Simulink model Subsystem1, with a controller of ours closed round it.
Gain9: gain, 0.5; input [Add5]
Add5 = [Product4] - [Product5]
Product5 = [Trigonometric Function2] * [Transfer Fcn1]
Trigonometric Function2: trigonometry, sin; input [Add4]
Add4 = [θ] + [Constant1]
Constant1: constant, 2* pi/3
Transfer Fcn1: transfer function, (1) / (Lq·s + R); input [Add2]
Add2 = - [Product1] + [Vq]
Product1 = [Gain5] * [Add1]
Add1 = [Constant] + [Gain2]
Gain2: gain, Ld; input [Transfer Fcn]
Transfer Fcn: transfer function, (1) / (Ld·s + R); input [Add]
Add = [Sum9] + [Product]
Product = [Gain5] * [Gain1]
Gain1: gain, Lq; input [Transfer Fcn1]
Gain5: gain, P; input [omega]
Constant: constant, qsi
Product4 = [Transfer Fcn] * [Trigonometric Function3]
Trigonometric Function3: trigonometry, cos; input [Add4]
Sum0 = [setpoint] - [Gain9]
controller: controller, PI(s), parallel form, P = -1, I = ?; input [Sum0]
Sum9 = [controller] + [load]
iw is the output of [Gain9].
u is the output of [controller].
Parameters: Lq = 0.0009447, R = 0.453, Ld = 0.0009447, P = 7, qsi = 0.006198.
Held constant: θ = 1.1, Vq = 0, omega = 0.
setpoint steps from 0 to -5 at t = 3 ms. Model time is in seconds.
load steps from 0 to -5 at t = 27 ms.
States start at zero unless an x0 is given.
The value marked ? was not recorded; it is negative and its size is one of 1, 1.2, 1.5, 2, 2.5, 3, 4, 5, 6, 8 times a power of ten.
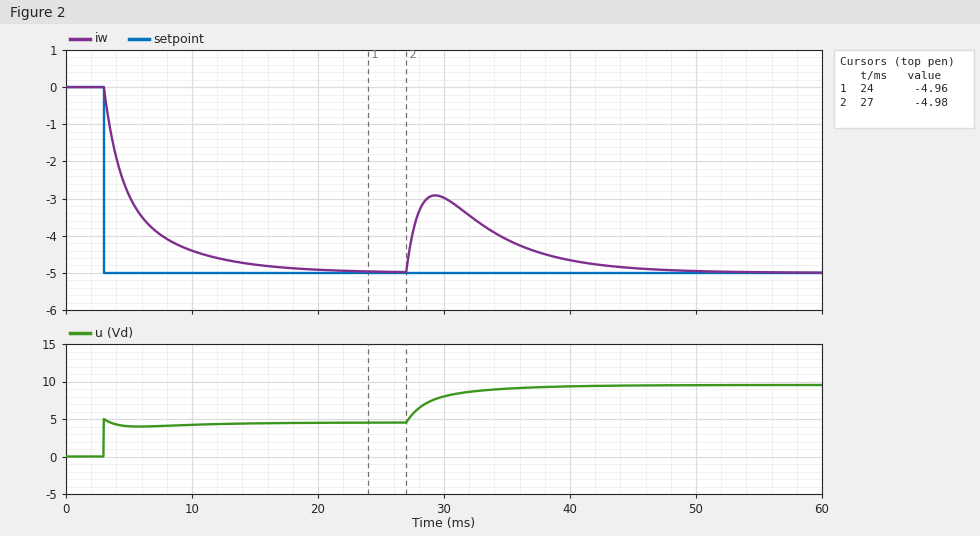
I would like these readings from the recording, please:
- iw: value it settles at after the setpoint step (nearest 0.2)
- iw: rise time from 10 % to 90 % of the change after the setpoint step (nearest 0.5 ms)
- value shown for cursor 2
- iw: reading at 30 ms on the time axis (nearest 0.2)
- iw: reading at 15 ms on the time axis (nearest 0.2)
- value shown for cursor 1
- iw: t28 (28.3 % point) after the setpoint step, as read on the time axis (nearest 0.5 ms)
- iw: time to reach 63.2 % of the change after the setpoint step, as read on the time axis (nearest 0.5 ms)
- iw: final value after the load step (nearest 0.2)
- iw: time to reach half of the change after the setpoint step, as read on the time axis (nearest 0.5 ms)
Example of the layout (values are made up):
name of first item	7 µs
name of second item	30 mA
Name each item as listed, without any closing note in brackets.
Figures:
iw: value it settles at after the setpoint step	-5.0
iw: rise time from 10 % to 90 % of the change after the setpoint step	7.5 ms
value shown for cursor 2	-4.98
iw: reading at 30 ms on the time axis	-3.0
iw: reading at 15 ms on the time axis	-4.8
value shown for cursor 1	-4.96
iw: t28 (28.3 % point) after the setpoint step, as read on the time axis	3.5 ms
iw: time to reach 63.2 % of the change after the setpoint step, as read on the time axis	5.5 ms
iw: final value after the load step	-5.0
iw: time to reach half of the change after the setpoint step, as read on the time axis	4.5 ms
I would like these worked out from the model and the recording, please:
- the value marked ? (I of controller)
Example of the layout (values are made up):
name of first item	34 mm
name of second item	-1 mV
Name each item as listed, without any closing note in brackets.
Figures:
the value marked ?	-300
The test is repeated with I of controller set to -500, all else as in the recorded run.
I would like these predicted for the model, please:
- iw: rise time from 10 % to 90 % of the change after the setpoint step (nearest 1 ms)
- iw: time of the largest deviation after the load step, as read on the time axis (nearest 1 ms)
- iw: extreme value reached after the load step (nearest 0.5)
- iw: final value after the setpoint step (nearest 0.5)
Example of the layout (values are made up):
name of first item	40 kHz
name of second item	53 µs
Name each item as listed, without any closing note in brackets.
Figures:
iw: rise time from 10 % to 90 % of the change after the setpoint step	4 ms
iw: time of the largest deviation after the load step, as read on the time axis	29 ms
iw: extreme value reached after the load step	-3.0
iw: final value after the setpoint step	-5.0
